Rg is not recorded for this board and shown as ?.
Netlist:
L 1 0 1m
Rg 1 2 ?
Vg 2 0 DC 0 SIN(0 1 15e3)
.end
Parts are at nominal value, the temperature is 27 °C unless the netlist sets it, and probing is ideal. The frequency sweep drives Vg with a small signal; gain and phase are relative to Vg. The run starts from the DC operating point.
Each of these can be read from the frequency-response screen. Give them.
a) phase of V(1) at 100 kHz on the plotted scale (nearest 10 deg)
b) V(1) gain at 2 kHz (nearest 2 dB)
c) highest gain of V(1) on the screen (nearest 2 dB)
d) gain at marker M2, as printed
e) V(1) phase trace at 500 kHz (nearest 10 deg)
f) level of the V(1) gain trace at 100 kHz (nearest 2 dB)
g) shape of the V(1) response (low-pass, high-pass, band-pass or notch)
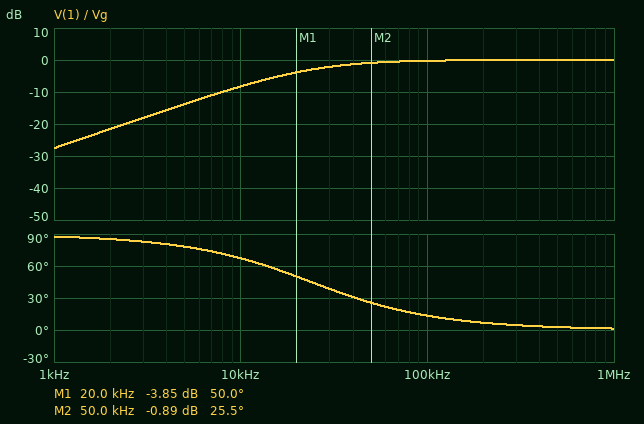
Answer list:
10 deg
-22 dB
0 dB
-0.89 dB
0 deg
0 dB
high-pass
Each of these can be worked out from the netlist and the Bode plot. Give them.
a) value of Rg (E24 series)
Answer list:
150 Ω
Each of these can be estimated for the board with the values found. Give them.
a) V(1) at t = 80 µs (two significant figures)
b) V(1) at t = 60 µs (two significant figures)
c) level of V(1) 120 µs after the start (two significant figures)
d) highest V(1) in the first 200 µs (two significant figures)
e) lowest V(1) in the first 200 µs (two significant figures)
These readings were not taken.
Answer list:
410 mV
200 mV
-130 mV
530 mV
-530 mV
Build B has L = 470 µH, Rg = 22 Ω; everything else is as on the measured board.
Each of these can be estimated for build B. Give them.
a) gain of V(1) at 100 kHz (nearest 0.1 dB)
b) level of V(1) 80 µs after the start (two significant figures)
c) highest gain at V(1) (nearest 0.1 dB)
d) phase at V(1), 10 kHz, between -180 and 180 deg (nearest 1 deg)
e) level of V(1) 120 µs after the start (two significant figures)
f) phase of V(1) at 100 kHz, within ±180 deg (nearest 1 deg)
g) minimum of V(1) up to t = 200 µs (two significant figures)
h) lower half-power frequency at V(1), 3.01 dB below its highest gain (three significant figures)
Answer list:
0 dB
880 mV
0 dB
37 deg
-640 mV
4 deg
-940 mV
7.45 kHz
